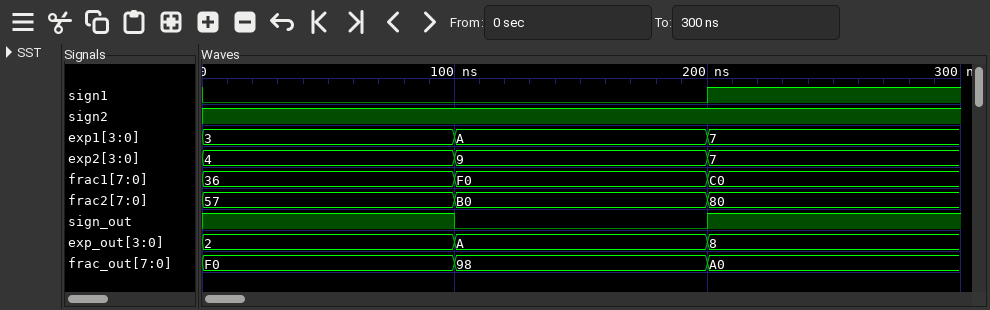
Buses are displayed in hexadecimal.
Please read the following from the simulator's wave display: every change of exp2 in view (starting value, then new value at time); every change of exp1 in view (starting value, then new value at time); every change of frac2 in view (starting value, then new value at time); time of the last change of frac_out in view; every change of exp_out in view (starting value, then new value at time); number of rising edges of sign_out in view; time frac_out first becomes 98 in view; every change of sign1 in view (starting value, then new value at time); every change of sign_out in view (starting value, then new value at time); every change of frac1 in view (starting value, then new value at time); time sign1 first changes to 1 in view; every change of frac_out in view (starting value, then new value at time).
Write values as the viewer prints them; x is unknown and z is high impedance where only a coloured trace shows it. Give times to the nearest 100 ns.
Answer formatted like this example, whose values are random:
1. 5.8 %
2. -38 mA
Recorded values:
1. 4, 9 at 100 ns, 7 at 200 ns
2. 3, A at 100 ns, 7 at 200 ns
3. 57, B0 at 100 ns, 80 at 200 ns
4. 200 ns
5. 2, A at 100 ns, 8 at 200 ns
6. 1
7. 100 ns
8. 0, 1 at 200 ns
9. 1, 0 at 100 ns, 1 at 200 ns
10. 36, F0 at 100 ns, C0 at 200 ns
11. 200 ns
12. F0, 98 at 100 ns, A0 at 200 ns
